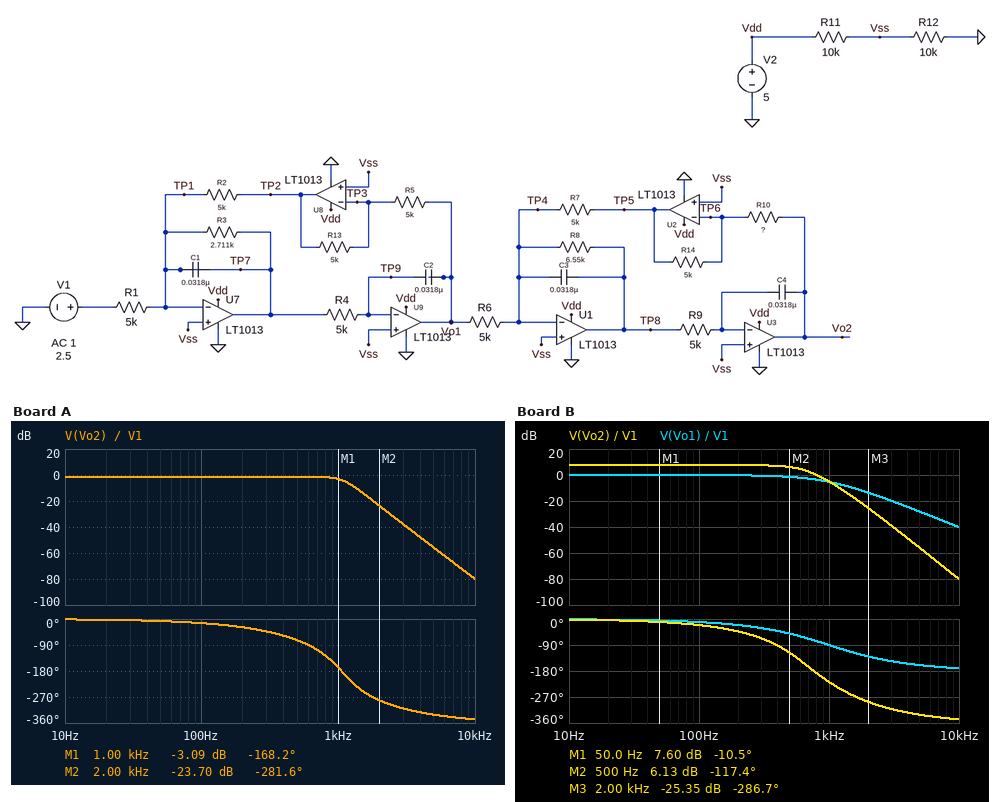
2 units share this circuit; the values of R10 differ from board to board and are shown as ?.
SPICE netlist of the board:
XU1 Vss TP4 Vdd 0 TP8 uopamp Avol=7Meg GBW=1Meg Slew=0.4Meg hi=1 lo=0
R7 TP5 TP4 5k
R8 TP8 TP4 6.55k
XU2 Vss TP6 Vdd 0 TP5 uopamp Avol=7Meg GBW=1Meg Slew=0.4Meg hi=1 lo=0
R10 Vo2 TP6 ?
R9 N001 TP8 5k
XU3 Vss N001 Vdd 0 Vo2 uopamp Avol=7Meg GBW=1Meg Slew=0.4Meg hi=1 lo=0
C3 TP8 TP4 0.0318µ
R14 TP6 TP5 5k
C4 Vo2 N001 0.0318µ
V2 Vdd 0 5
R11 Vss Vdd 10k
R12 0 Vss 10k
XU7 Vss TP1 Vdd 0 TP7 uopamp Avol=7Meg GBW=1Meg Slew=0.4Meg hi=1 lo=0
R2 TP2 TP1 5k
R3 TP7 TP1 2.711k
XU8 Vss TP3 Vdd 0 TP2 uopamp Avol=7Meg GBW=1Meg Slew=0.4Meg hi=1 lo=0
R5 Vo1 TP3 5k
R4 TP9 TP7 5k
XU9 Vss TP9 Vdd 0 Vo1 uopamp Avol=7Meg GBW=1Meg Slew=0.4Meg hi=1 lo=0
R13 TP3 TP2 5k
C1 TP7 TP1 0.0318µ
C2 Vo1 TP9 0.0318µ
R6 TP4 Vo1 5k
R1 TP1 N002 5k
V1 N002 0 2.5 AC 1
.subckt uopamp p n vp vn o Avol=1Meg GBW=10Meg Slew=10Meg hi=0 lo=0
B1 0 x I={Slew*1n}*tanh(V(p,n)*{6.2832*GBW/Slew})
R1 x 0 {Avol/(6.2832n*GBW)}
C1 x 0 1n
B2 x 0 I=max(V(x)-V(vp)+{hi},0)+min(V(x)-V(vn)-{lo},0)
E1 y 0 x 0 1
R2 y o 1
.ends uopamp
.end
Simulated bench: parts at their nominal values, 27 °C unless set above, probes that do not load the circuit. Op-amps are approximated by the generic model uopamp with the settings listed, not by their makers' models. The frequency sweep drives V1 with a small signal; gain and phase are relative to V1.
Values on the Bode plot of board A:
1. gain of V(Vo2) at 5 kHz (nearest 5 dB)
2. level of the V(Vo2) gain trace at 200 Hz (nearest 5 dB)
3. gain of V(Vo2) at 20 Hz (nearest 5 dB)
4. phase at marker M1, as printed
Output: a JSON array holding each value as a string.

["-55 dB", "0 dB", "0 dB", "-168.2 deg"]
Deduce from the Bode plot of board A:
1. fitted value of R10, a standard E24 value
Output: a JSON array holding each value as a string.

["4.3 kΩ"]
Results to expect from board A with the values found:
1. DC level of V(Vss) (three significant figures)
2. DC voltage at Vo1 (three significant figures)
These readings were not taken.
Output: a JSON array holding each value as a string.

["2.50 V", "2.50 V"]
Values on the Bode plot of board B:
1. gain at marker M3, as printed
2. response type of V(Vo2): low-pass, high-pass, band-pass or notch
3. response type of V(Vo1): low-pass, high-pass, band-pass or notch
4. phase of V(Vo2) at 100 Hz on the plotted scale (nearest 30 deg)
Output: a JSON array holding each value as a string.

["-25.35 dB", "low-pass", "low-pass", "-30 deg"]
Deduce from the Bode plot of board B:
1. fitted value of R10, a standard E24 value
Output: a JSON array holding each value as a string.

["12 kΩ"]
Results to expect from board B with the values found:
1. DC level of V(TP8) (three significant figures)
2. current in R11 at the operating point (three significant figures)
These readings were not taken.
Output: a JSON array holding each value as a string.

["2.50 V", "250 µA"]
